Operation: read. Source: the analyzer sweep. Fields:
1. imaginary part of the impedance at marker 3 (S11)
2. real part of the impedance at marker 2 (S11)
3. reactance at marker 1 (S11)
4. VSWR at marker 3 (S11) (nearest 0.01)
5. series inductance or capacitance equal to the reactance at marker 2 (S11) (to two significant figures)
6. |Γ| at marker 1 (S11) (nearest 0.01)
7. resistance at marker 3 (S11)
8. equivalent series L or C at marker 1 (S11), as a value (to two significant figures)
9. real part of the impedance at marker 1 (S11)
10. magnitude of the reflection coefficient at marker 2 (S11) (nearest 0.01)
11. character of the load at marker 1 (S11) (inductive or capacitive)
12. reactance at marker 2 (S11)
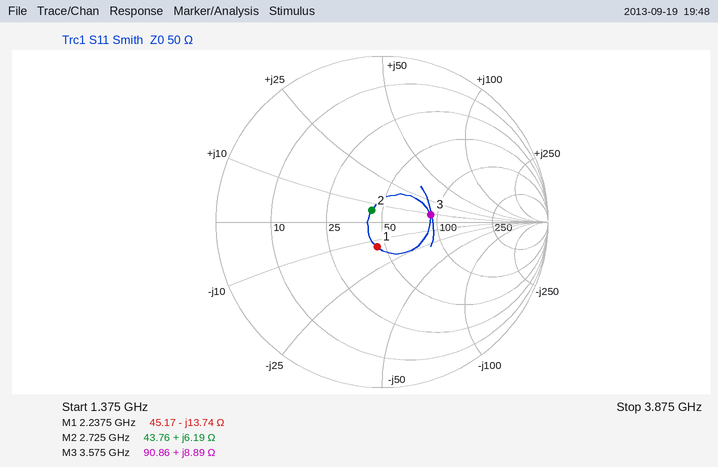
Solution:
+8.89 Ω
43.76 Ω
-13.74 Ω
1.84
360 pH
0.15
90.86 Ω
5.2 pF
45.17 Ω
0.09
capacitive
+6.19 Ω
